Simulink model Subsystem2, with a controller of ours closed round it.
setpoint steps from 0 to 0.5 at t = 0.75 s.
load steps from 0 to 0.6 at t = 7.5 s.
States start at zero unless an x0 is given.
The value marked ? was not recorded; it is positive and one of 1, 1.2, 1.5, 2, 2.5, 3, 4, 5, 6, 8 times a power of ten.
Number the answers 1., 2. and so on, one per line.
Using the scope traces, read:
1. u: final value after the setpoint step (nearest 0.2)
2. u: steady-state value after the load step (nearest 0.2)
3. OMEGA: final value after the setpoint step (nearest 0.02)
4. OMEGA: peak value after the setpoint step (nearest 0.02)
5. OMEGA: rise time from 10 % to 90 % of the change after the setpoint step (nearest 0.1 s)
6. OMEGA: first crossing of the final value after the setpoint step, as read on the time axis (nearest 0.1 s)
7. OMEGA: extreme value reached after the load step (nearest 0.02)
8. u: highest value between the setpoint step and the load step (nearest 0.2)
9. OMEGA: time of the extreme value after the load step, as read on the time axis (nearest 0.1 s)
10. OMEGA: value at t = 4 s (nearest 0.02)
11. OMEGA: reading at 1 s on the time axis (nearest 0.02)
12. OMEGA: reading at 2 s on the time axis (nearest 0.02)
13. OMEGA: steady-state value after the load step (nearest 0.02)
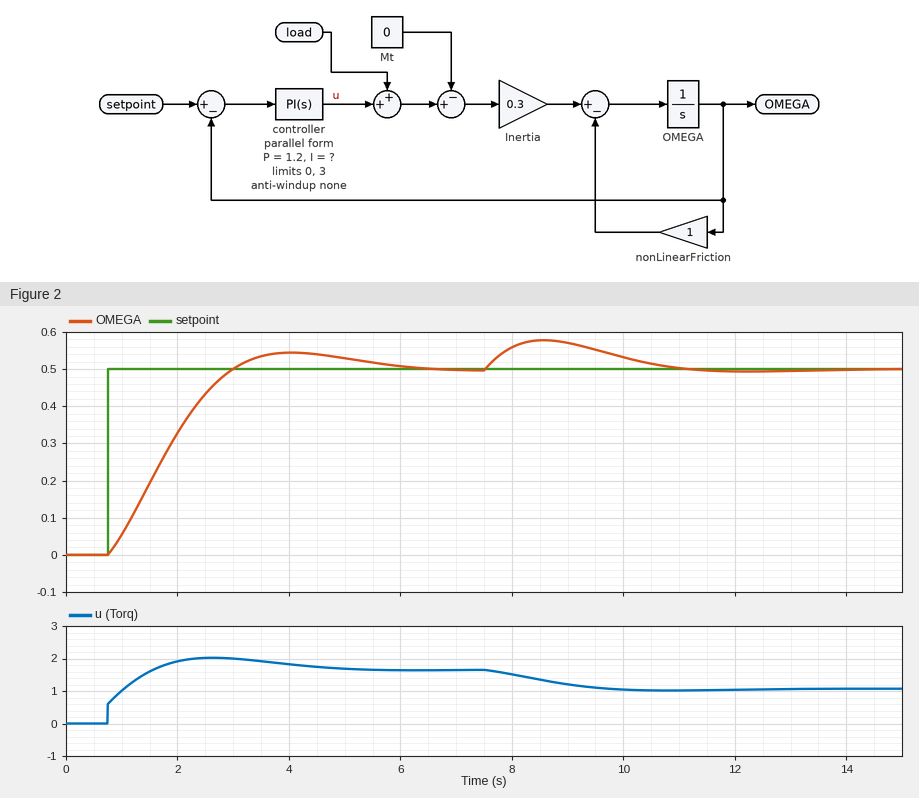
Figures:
1. 1.6
2. 1.0
3. 0.50
4. 0.54
5. 1.6 s
6. 3.0 s
7. 0.58
8. 2.0
9. 8.6 s
10. 0.54
11. 0.06
12. 0.32
13. 0.50
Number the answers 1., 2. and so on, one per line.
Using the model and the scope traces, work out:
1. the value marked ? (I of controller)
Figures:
1. 4
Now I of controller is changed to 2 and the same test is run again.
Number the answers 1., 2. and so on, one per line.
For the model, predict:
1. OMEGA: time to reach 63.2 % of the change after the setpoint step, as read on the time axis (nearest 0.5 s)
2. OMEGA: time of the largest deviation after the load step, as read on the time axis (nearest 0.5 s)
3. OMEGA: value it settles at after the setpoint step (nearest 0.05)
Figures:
1. 2.5 s
2. 9.0 s
3. 0.50
